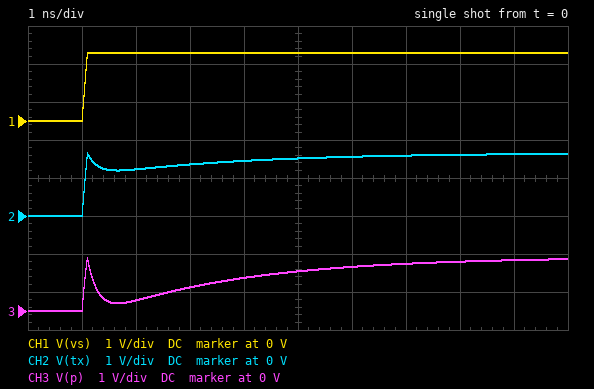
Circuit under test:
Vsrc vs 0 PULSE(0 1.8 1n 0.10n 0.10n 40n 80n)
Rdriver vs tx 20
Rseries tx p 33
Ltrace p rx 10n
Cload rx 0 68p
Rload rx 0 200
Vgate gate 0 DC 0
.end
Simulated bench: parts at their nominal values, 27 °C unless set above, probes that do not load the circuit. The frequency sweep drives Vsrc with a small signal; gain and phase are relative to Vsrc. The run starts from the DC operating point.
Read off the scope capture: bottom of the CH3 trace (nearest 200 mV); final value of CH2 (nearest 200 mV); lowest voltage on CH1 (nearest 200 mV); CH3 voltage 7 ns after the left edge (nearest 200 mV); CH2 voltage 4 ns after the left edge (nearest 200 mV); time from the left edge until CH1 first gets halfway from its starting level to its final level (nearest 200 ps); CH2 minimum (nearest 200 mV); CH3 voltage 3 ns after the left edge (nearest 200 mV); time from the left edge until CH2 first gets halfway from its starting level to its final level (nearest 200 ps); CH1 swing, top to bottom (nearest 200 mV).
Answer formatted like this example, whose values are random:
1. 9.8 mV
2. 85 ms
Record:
1. 0 V
2. 1.6 V
3. 0 V
4. 1.2 V
5. 1.4 V
6. 1.0 ns
7. 0 V
8. 600 mV
9. 1.0 ns
10. 1.8 V
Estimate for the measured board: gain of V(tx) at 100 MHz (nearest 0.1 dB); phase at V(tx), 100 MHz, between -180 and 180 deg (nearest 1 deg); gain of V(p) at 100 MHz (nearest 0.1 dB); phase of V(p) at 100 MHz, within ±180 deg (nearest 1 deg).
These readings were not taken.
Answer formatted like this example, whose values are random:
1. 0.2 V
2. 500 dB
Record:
1. -3.4 dB
2. -8 deg
3. -10.7 dB
4. -64 deg
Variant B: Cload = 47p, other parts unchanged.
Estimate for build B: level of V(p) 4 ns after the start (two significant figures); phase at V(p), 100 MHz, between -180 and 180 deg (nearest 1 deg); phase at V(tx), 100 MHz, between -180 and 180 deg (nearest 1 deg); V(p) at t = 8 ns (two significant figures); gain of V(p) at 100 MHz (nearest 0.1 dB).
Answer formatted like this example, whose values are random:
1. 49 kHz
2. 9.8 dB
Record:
1. 1.1 V
2. -54 deg
3. -10 deg
4. 1.4 V
5. -7.5 dB
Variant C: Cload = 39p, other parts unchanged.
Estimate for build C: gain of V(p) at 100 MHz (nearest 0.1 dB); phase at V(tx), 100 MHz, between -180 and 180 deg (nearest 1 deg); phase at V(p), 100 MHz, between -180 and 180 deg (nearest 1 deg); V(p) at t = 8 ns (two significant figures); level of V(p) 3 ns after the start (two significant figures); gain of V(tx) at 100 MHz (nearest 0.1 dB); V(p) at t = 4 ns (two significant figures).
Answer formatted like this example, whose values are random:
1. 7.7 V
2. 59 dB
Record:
1. -6.2 dB
2. -10 deg
3. -48 deg
4. 1.4 V
5. 920 mV
6. -2.4 dB
7. 1.2 V
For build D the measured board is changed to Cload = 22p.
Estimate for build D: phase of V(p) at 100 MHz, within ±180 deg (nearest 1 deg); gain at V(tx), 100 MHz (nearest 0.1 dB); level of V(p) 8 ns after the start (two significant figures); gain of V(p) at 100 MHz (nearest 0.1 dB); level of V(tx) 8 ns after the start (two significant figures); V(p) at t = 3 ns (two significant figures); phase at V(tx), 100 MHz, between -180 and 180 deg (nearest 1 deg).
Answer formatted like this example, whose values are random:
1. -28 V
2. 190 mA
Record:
1. -31 deg
2. -1.5 dB
3. 1.4 V
4. -3.7 dB
5. 1.7 V
6. 1.2 V
7. -9 deg
